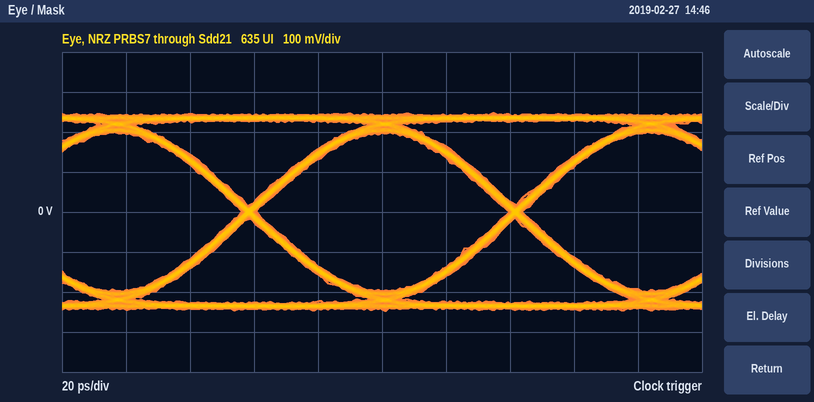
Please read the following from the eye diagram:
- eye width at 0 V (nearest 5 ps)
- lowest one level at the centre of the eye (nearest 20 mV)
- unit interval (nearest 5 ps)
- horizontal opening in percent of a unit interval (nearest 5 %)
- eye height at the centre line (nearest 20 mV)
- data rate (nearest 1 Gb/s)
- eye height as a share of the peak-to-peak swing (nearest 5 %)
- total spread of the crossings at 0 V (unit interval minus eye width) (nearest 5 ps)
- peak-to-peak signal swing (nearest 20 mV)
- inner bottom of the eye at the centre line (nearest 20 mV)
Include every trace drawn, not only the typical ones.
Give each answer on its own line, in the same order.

80 ps
200 mV
85 ps
95 %
400 mV
12 Gb/s
80 %
5 ps
500 mV
-200 mV
